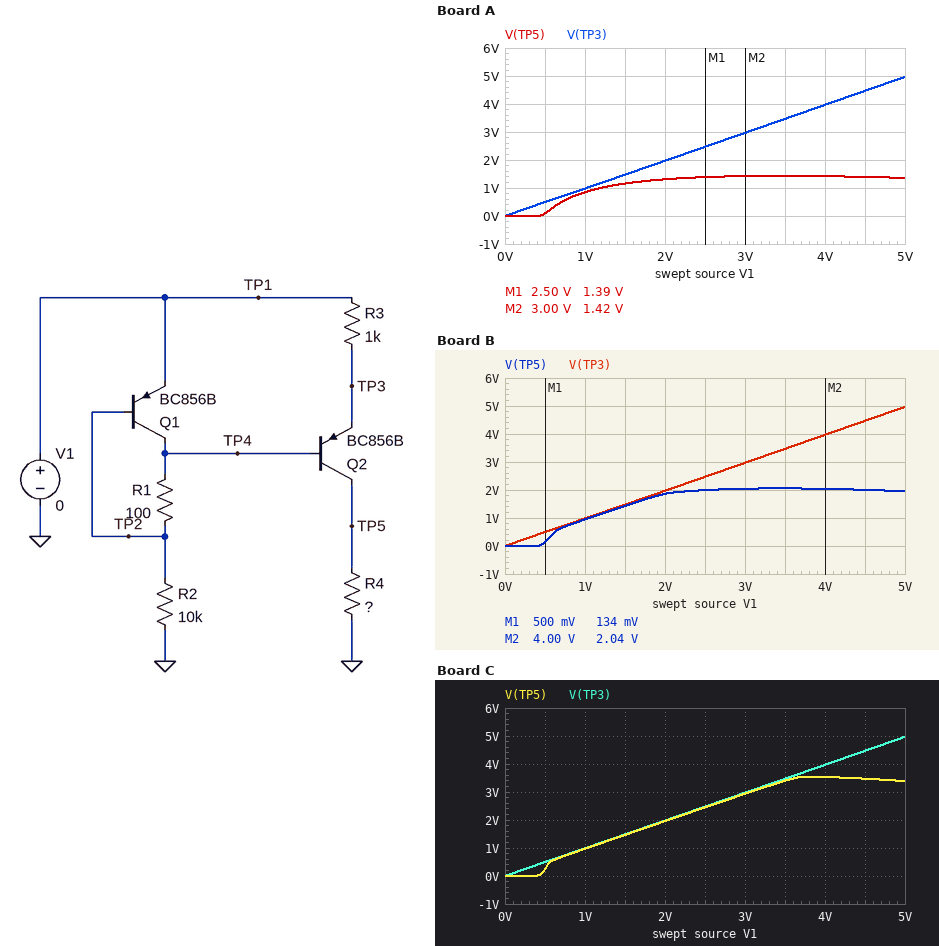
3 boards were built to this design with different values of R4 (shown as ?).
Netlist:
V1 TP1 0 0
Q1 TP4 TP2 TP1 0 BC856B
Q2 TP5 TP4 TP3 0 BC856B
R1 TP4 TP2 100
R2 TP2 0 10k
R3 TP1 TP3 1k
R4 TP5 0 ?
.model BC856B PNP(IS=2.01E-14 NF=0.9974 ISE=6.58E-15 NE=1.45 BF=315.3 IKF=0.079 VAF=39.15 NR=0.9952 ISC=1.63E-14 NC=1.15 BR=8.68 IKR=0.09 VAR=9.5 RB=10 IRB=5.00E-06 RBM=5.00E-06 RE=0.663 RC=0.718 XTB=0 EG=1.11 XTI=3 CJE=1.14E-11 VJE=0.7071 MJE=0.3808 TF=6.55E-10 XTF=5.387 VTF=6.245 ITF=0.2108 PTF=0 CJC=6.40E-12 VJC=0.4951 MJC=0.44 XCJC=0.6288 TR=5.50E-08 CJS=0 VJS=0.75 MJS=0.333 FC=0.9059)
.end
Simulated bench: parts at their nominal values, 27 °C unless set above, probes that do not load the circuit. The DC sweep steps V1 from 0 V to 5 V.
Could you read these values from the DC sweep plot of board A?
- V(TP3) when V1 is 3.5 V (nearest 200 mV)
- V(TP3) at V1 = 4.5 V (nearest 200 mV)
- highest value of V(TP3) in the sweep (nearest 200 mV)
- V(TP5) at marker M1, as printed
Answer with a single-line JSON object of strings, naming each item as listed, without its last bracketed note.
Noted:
{"V(TP3) when V1 is 3.5 V": "3.4 V", "V(TP3) at V1 = 4.5 V": "4.4 V", "highest value of V(TP3) in the sweep": "5.0 V", "V(TP5) at marker M1, as printed": "1.39 V"}
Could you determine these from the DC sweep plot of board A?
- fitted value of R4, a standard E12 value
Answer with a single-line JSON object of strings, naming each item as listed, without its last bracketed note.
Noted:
{"fitted value of R4, a standard E12 value": "47 kΩ"}
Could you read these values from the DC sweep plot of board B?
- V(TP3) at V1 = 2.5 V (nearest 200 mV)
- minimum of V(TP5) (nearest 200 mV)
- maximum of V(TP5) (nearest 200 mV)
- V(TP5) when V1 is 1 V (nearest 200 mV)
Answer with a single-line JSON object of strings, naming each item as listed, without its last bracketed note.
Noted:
{"V(TP3) at V1 = 2.5 V": "2.4 V", "minimum of V(TP5)": "0 V", "maximum of V(TP5)": "2.0 V", "V(TP5) when V1 is 1 V": "1.0 V"}
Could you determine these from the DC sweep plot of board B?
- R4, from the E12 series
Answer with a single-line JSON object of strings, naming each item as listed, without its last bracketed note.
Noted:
{"R4, from the E12 series": "68 kΩ"}
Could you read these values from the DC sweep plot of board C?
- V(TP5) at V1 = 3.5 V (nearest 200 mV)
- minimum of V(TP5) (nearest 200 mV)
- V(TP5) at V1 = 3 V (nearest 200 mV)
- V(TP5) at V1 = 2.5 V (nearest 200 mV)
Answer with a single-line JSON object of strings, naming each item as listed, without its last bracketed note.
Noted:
{"V(TP5) at V1 = 3.5 V": "3.4 V", "minimum of V(TP5)": "0 V", "V(TP5) at V1 = 3 V": "3.0 V", "V(TP5) at V1 = 2.5 V": "2.4 V"}
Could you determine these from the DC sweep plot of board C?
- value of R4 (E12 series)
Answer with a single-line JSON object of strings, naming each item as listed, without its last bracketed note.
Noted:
{"value of R4": "120 kΩ"}
